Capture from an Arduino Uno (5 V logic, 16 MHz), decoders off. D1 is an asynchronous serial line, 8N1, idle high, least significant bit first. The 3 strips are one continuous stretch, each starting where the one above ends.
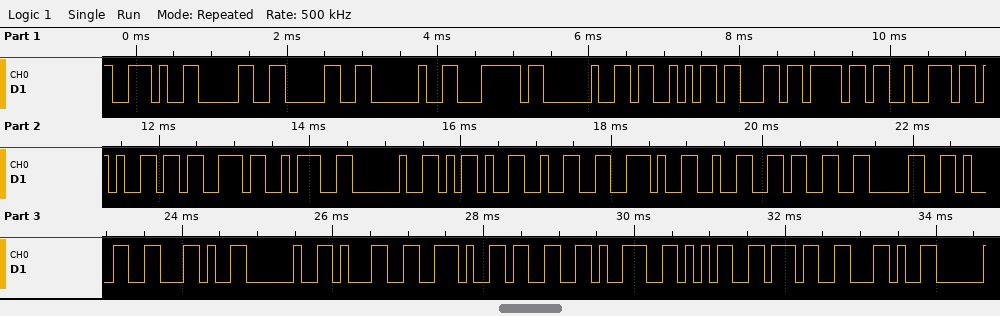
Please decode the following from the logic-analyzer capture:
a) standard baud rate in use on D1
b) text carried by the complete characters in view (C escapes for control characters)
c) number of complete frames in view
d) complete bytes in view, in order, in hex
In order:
9600 baud
".00 | Scores: -2.2301, 1.3957,"
30
0x2E 0x30 0x30 0x20 0x7C 0x20 0x53 0x63 0x6F 0x72 0x65 0x73 0x3A 0x20 0x2D 0x32 0x2E 0x32 0x33 0x30 0x31 0x2C 0x20 0x31 0x2E 0x33 0x39 0x35 0x37 0x2C
